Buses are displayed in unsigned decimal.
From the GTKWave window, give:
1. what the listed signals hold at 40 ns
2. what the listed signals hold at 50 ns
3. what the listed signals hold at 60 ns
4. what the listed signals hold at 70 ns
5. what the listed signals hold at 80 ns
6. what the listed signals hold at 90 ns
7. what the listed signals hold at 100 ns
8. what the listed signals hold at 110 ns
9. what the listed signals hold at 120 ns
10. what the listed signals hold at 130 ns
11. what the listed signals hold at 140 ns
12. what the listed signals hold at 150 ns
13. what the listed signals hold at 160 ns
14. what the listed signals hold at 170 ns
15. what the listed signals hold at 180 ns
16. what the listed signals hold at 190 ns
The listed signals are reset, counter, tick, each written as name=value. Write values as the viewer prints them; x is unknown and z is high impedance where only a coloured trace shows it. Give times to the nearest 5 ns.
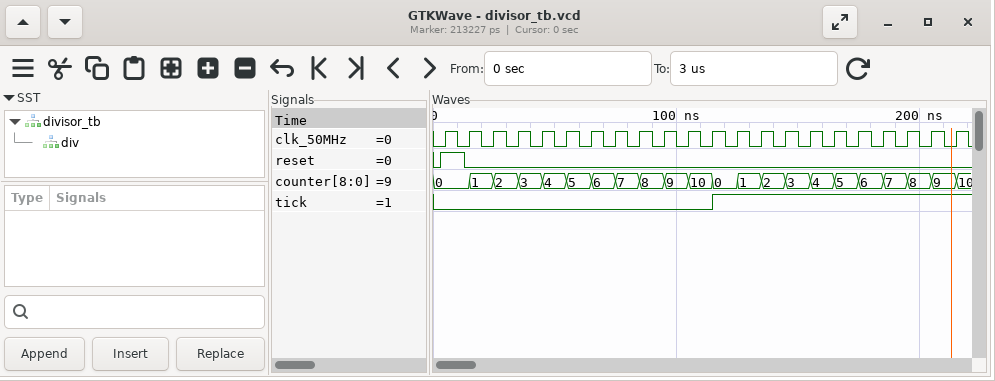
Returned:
reset=0, counter=3, tick=0
reset=0, counter=4, tick=0
reset=0, counter=5, tick=0
reset=0, counter=6, tick=0
reset=0, counter=7, tick=0
reset=0, counter=8, tick=0
reset=0, counter=9, tick=0
reset=0, counter=10, tick=0
reset=0, counter=0, tick=1
reset=0, counter=1, tick=1
reset=0, counter=2, tick=1
reset=0, counter=3, tick=1
reset=0, counter=4, tick=1
reset=0, counter=5, tick=1
reset=0, counter=6, tick=1
reset=0, counter=7, tick=1
